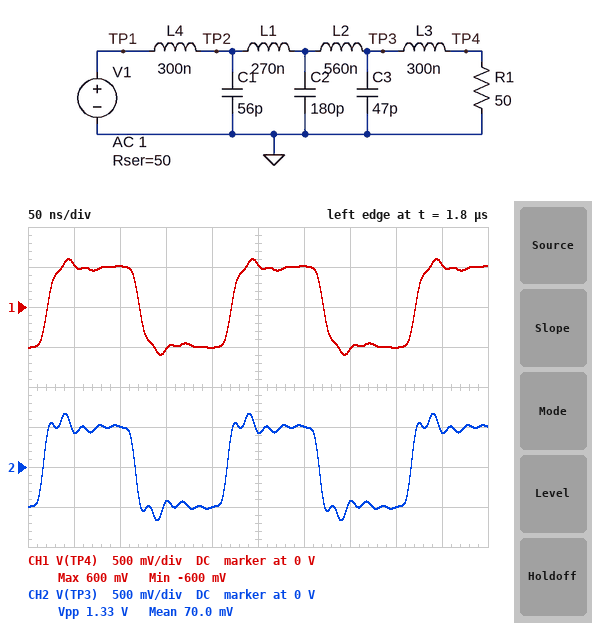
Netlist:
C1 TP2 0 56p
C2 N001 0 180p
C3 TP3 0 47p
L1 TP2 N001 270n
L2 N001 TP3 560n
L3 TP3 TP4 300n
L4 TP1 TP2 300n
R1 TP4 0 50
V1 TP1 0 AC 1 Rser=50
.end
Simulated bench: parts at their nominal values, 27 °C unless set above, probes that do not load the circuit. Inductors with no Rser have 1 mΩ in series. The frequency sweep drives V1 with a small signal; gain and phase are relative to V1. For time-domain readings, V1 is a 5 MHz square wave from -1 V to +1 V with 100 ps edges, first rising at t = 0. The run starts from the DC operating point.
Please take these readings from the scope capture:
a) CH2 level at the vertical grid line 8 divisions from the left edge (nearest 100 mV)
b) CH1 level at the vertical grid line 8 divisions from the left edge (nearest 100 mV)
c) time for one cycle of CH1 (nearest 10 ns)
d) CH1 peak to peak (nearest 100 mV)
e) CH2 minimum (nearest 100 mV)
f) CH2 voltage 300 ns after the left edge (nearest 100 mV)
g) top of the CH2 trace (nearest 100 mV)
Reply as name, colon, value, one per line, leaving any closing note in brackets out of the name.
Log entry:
CH2 level at the vertical grid line 8 divisions from the left edge: -500 mV
CH1 level at the vertical grid line 8 divisions from the left edge: -500 mV
time for one cycle of CH1: 200 ns
CH1 peak to peak: 1.2 V
CH2 minimum: -700 mV
CH2 voltage 300 ns after the left edge: 500 mV
top of the CH2 trace: 700 mV
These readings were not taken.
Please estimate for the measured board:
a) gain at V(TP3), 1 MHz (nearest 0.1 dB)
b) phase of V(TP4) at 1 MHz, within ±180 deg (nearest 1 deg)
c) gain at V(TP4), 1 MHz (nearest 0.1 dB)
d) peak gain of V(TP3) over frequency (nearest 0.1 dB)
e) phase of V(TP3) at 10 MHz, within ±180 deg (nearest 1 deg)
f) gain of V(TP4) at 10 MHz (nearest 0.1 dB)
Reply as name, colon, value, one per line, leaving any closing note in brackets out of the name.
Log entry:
gain at V(TP3), 1 MHz: -6.0 dB
phase of V(TP4) at 1 MHz, within ±180 deg: -8 deg
gain at V(TP4), 1 MHz: -6.0 dB
peak gain of V(TP3) over frequency: -5.1 dB
phase of V(TP3) at 10 MHz, within ±180 deg: -54 deg
gain of V(TP4) at 10 MHz: -6.3 dB
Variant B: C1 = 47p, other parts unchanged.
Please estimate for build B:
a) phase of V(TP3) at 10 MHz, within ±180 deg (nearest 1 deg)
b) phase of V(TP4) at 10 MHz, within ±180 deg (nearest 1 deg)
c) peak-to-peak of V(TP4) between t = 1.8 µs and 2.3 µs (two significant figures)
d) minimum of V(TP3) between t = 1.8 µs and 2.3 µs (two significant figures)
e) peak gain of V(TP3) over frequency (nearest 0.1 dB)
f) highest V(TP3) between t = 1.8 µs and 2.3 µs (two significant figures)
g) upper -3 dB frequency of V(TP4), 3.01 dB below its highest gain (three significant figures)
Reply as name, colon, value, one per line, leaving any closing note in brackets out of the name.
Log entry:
phase of V(TP3) at 10 MHz, within ±180 deg: -53 deg
phase of V(TP4) at 10 MHz, within ±180 deg: -74 deg
peak-to-peak of V(TP4) between t = 1.8 µs and 2.3 µs: 1.2 V
minimum of V(TP3) between t = 1.8 µs and 2.3 µs: -650 mV
peak gain of V(TP3) over frequency: -5.0 dB
highest V(TP3) between t = 1.8 µs and 2.3 µs: 650 mV
upper -3 dB frequency of V(TP4), 3.01 dB below its highest gain: 21.8 MHz
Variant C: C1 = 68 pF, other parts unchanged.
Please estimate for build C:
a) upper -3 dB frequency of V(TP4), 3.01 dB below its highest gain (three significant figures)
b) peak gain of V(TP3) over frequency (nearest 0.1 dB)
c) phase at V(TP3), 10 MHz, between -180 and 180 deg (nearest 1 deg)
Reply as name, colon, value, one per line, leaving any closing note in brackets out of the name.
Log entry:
upper -3 dB frequency of V(TP4), 3.01 dB below its highest gain: 21.5 MHz
peak gain of V(TP3) over frequency: -3.3 dB
phase at V(TP3), 10 MHz, between -180 and 180 deg: -56 deg
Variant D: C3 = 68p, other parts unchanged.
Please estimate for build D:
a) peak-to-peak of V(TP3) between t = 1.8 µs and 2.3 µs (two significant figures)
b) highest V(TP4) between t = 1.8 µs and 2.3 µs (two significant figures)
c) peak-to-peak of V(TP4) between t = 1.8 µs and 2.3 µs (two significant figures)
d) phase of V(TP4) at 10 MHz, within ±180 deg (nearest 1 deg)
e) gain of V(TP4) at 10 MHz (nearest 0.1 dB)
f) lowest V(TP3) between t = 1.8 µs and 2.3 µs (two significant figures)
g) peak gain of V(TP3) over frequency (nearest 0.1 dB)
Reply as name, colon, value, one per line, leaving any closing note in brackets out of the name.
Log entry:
peak-to-peak of V(TP3) between t = 1.8 µs and 2.3 µs: 1.2 V
highest V(TP4) between t = 1.8 µs and 2.3 µs: 560 mV
peak-to-peak of V(TP4) between t = 1.8 µs and 2.3 µs: 1.1 V
phase of V(TP4) at 10 MHz, within ±180 deg: -77 deg
gain of V(TP4) at 10 MHz: -6.2 dB
lowest V(TP3) between t = 1.8 µs and 2.3 µs: -620 mV
peak gain of V(TP3) over frequency: -5.0 dB
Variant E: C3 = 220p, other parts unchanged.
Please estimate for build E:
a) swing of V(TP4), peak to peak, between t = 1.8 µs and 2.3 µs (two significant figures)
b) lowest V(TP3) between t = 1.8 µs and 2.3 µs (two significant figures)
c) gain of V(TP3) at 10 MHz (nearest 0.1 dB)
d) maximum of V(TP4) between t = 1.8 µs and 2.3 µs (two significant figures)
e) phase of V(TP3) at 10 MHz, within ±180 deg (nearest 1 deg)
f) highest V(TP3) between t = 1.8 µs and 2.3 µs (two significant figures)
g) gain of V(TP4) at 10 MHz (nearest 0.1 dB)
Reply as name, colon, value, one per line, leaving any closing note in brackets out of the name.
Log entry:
swing of V(TP4), peak to peak, between t = 1.8 µs and 2.3 µs: 1.3 V
lowest V(TP3) between t = 1.8 µs and 2.3 µs: -730 mV
gain of V(TP3) at 10 MHz: -5.5 dB
maximum of V(TP4) between t = 1.8 µs and 2.3 µs: 650 mV
phase of V(TP3) at 10 MHz, within ±180 deg: -73 deg
highest V(TP3) between t = 1.8 µs and 2.3 µs: 730 mV
gain of V(TP4) at 10 MHz: -6.1 dB
